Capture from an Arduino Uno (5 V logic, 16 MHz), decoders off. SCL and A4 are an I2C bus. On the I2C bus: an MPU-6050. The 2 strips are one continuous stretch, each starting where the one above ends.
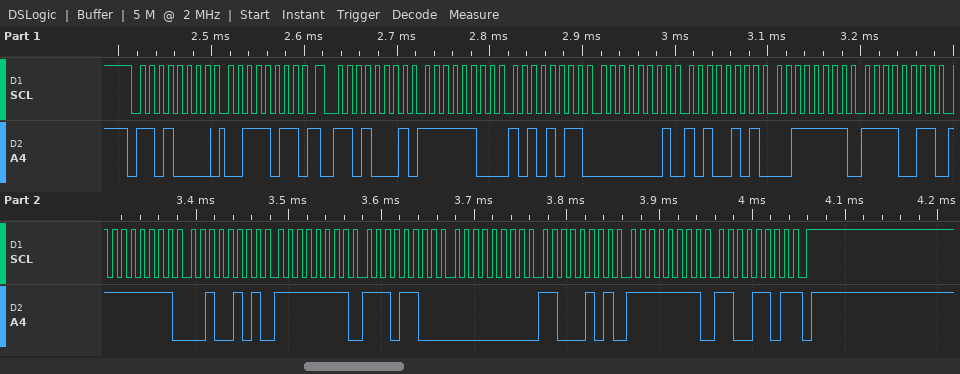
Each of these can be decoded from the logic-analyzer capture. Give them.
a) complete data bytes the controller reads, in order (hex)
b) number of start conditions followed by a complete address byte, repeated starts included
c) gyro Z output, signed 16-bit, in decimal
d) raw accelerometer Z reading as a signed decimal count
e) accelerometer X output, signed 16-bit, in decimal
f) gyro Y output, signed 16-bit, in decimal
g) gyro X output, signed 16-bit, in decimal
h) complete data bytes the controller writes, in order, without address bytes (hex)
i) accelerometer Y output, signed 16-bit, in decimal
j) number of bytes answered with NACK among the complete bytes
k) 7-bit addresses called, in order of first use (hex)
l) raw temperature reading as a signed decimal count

FC AB 01 A5 3F F3 FF 25 FF EC 00 C5 FF CD
2
-51
16371
-853
197
-20
3B
421
1
0x68
-219
